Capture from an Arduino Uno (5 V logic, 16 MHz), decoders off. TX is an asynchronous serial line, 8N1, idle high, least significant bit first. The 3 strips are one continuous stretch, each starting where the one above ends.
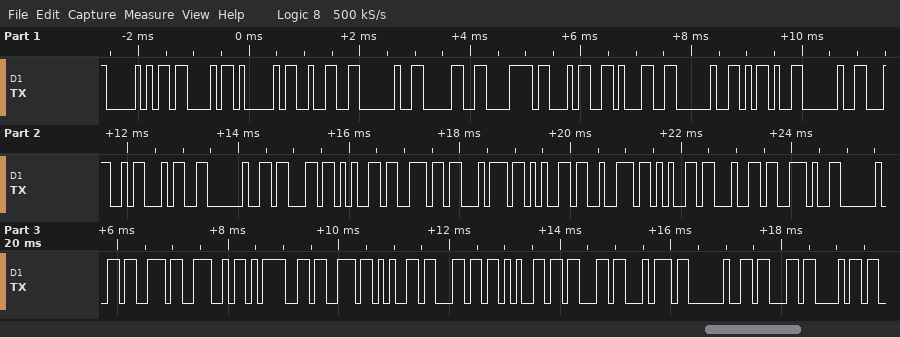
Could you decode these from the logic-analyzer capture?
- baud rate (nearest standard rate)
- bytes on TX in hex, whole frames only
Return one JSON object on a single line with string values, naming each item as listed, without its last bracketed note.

{"baud rate": "9600 baud", "bytes on TX in hex, whole frames only": "50 43 41 32 20 30 78 34 31 20 2D 20 4C 34 20 63 65 6E 74 65 72 65 64 2E 20 73 4E 3D 73 65 6C 65 63 74 20 63 68"}
